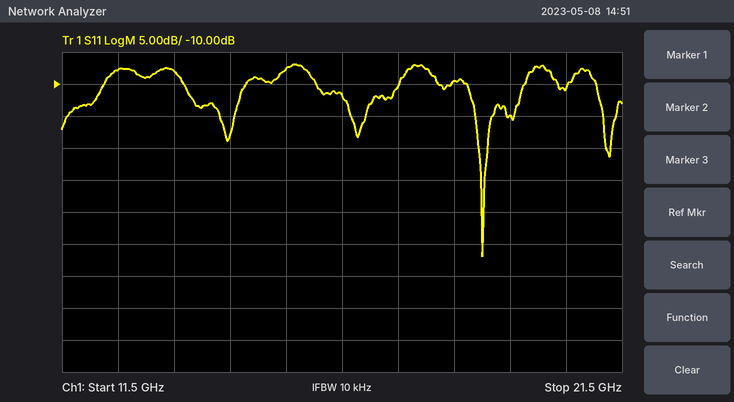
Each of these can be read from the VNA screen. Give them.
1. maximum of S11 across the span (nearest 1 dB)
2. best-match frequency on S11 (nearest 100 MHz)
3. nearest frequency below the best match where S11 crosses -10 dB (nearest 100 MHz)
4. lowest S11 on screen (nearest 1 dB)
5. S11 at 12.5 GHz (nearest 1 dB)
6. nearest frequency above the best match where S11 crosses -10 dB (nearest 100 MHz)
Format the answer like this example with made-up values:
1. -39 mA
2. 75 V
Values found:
1. -7 dB
2. 19.0 GHz
3. 18.7 GHz
4. -37 dB
5. -8 dB
6. 19.8 GHz
